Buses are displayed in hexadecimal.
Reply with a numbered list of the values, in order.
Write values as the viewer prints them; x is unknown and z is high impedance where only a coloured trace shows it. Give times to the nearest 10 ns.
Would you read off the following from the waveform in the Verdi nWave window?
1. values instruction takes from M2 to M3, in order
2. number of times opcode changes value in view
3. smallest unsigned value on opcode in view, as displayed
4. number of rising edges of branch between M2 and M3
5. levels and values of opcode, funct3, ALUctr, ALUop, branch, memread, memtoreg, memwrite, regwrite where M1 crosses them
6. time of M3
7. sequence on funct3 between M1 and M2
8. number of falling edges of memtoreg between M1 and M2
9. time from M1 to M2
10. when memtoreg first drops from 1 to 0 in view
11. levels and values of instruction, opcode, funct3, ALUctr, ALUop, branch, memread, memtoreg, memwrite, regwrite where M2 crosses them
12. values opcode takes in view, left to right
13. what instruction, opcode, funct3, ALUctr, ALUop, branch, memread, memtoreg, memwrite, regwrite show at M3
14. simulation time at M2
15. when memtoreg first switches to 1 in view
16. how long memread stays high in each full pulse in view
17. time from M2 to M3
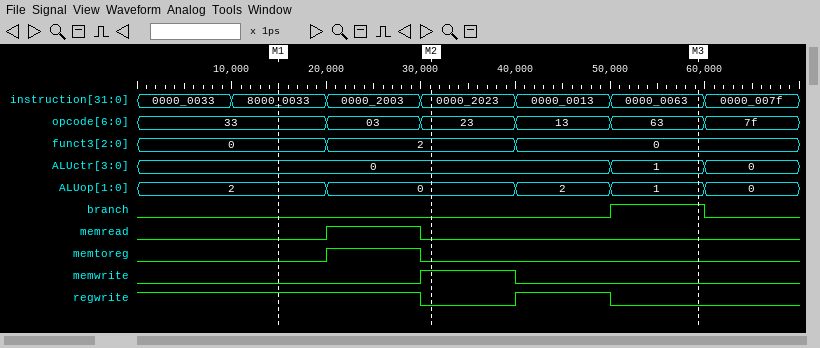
1. 0000_2023, 0000_0013, 0000_0063
2. 5
3. 03
4. 1
5. opcode=33, funct3=0, ALUctr=0, ALUop=2, branch=0, memread=0, memtoreg=0, memwrite=0, regwrite=1
6. 60 ns
7. 0, 2
8. 1
9. 20 ns
10. 30 ns
11. instruction=0000_2023, opcode=23, funct3=2, ALUctr=0, ALUop=0, branch=0, memread=0, memtoreg=0, memwrite=1, regwrite=0
12. 33, 03, 23, 13, 63, 7f
13. instruction=0000_0063, opcode=63, funct3=0, ALUctr=1, ALUop=1, branch=1, memread=0, memtoreg=0, memwrite=0, regwrite=0
14. 30 ns
15. 20 ns
16. 10 ns
17. 30 ns
